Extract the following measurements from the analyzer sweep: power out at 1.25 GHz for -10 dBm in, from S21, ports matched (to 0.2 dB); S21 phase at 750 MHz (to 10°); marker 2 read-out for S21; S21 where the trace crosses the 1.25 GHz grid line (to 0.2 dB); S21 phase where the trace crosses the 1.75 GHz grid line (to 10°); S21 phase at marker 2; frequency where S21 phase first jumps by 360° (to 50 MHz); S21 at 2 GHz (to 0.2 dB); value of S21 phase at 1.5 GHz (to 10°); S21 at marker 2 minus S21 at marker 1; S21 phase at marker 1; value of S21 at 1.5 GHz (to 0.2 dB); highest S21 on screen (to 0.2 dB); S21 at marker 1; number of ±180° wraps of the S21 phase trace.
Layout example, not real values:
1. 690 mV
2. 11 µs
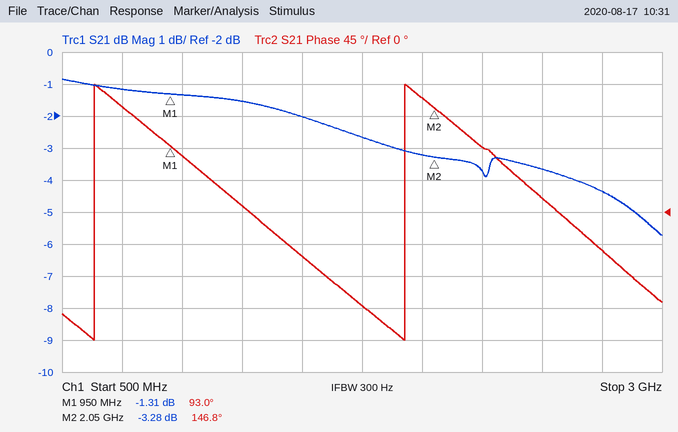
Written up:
1. -11.6 dBm
2. 150°
3. -3.28 dB
4. -1.6 dB
5. -130°
6. 146.8°
7. 650 MHz
8. -3.2 dB
9. -60°
10. -1.97 dB
11. 93.0°
12. -2.0 dB
13. -0.8 dB
14. -1.31 dB
15. 2
